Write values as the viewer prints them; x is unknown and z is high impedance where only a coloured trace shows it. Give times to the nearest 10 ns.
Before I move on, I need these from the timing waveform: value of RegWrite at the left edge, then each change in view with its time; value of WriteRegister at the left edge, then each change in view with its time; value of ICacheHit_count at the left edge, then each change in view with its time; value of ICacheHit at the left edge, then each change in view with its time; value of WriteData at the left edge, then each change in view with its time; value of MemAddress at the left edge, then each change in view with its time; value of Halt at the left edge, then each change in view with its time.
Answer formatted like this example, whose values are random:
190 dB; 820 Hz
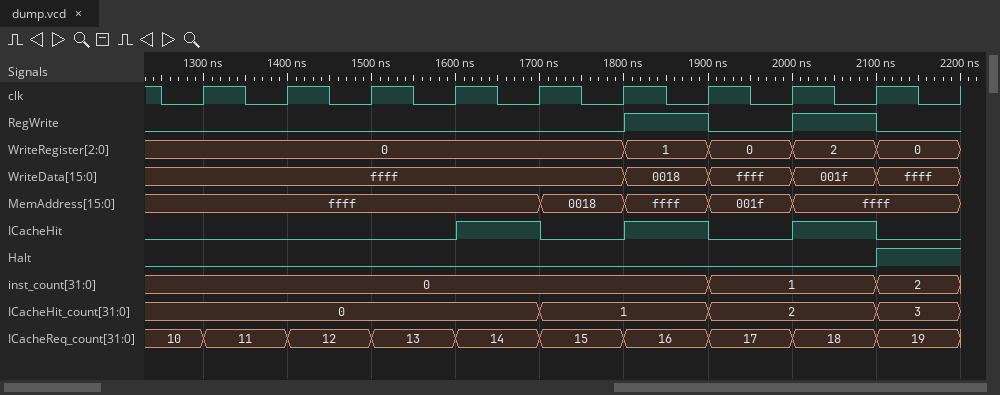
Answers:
0, 1 at 1800 ns, 0 at 1900 ns, 1 at 2000 ns, 0 at 2100 ns; 0, 1 at 1800 ns, 0 at 1900 ns, 2 at 2000 ns, 0 at 2100 ns; 0, 1 at 1700 ns, 2 at 1900 ns, 3 at 2100 ns; 0, 1 at 1600 ns, 0 at 1700 ns, 1 at 1800 ns, 0 at 1900 ns, 1 at 2000 ns, 0 at 2100 ns; ffff, 0018 at 1800 ns, ffff at 1900 ns, 001f at 2000 ns, ffff at 2100 ns; ffff, 0018 at 1700 ns, ffff at 1800 ns, 001f at 1900 ns, ffff at 2000 ns; 0, 1 at 2100 ns
